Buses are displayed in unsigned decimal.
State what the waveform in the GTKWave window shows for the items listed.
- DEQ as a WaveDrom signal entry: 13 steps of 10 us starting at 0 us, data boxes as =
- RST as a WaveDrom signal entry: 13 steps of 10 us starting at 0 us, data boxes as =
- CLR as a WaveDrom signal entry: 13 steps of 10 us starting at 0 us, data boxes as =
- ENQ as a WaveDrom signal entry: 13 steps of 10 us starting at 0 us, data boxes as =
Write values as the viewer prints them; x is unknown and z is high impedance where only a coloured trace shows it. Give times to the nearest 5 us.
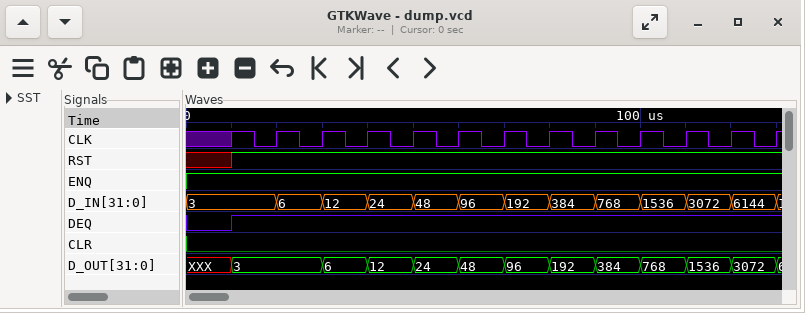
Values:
{name: 'DEQ', wave: '01...........'}
{name: 'RST', wave: 'x1...........'}
{name: 'CLR', wave: '0............'}
{name: 'ENQ', wave: '1............'}
